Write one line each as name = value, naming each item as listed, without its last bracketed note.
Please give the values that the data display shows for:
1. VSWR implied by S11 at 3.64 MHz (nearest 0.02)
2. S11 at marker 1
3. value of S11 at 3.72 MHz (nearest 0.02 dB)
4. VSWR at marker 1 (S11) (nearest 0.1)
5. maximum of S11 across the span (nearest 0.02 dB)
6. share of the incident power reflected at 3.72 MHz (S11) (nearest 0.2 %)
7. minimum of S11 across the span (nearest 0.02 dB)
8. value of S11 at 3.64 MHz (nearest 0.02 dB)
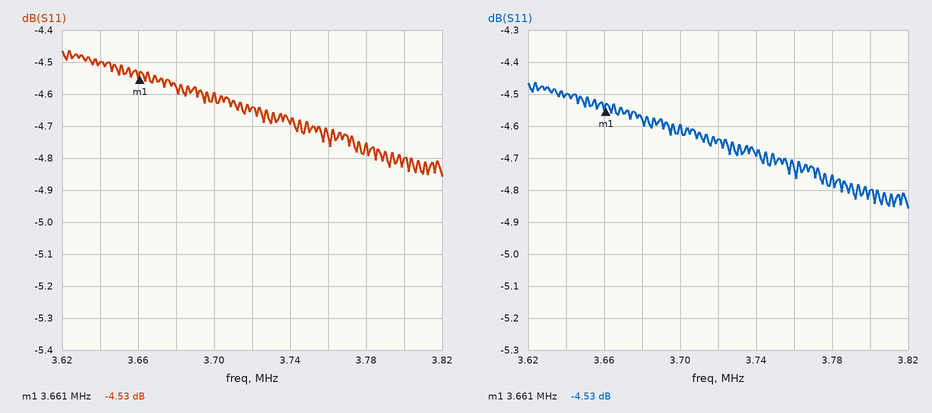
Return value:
VSWR implied by S11 at 3.64 MHz = 3.94
S11 at marker 1 = -4.53 dB
value of S11 at 3.72 MHz = -4.64 dB
VSWR at marker 1 (S11) = 3.9
maximum of S11 across the span = -4.46 dB
share of the incident power reflected at 3.72 MHz (S11) = 34.4 %
minimum of S11 across the span = -4.86 dB
value of S11 at 3.64 MHz = -4.50 dB
